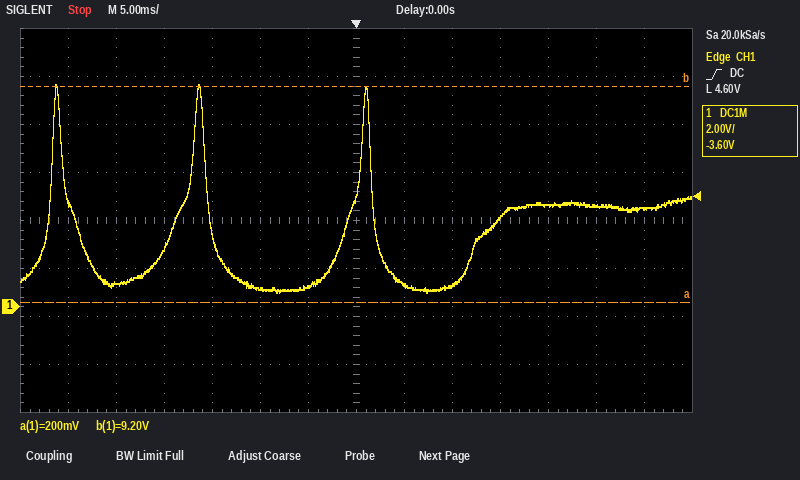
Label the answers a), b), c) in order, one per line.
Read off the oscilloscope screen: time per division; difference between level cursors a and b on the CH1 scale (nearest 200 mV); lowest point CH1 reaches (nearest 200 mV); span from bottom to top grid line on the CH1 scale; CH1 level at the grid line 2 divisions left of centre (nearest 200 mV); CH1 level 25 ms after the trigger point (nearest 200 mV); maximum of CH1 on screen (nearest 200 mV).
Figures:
a) 5 ms
b) 9.0 V
c) 600 mV
d) 16 V
e) 800 mV
f) 4.2 V
g) 9.2 V
